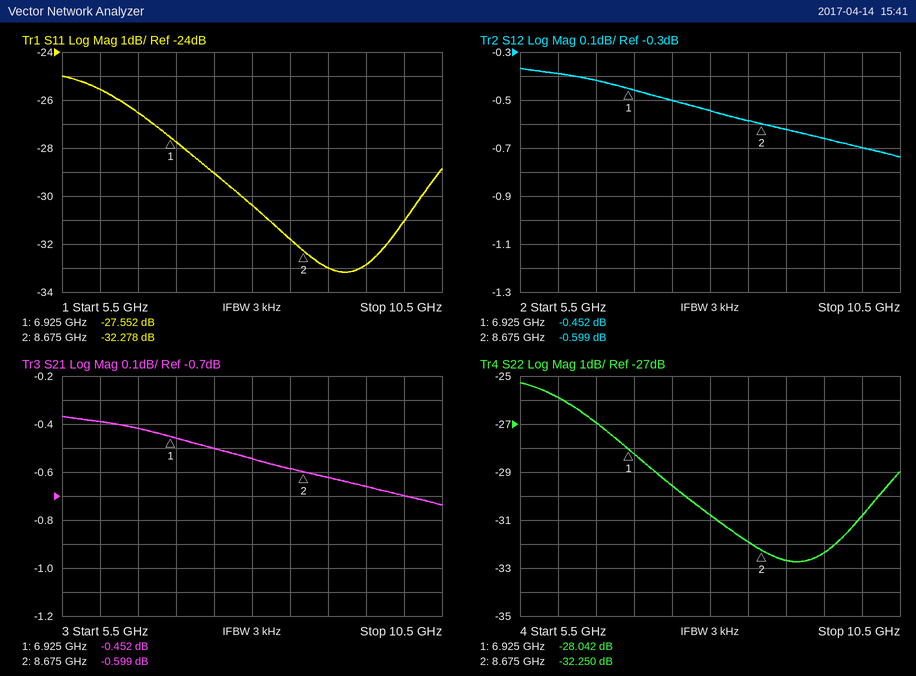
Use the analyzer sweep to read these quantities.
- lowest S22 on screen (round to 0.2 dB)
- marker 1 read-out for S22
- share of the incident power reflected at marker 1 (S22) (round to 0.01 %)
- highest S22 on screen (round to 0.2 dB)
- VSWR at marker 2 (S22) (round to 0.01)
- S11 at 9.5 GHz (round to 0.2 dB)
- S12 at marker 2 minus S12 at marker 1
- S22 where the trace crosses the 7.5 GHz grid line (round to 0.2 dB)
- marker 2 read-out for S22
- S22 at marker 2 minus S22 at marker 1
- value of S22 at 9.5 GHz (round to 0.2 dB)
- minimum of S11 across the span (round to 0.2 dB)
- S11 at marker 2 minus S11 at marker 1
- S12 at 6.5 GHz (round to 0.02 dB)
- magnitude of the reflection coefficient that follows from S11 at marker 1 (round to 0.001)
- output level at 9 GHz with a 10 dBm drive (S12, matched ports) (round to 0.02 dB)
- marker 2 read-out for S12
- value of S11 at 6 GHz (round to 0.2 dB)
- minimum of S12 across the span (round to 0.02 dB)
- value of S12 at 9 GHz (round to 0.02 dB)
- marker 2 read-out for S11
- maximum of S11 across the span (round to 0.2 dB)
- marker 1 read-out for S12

-32.8 dB
-28.042 dB
0.16 %
-25.2 dB
1.05
-32.8 dB
-0.147 dB
-29.6 dB
-32.250 dB
-4.208 dB
-32.4 dB
-33.2 dB
-4.726 dB
-0.42 dB
0.042
9.38 dBm
-0.599 dB
-25.6 dB
-0.74 dB
-0.62 dB
-32.278 dB
-25.0 dB
-0.452 dB
